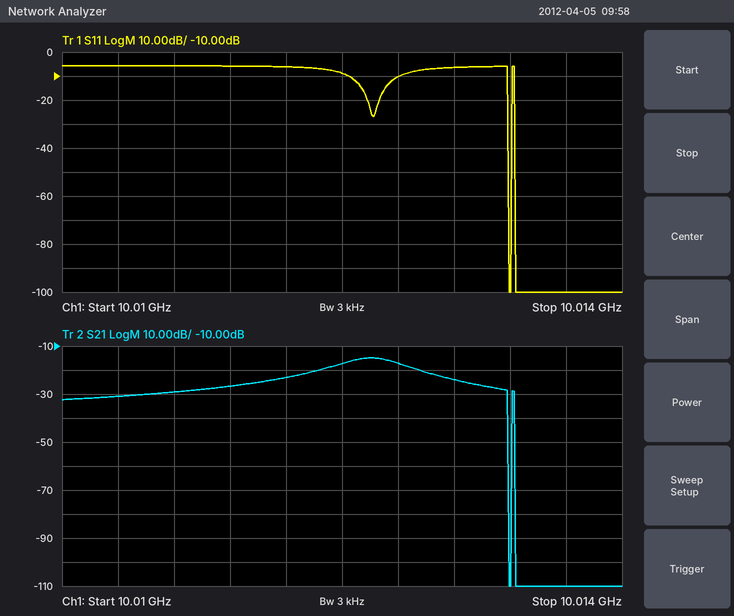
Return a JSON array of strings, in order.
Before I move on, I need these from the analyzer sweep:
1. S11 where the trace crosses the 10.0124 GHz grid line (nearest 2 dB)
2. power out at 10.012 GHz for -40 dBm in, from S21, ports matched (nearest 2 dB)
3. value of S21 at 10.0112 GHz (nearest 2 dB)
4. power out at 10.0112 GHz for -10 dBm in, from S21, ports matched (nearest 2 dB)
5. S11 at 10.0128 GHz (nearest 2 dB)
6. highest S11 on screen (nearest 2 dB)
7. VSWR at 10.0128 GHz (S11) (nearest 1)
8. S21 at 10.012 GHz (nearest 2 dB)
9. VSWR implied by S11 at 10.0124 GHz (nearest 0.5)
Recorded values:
["-10 dB", "-58 dBm", "-26 dB", "-36 dBm", "-6 dB", "-6 dB", "3", "-18 dB", "2.0"]
